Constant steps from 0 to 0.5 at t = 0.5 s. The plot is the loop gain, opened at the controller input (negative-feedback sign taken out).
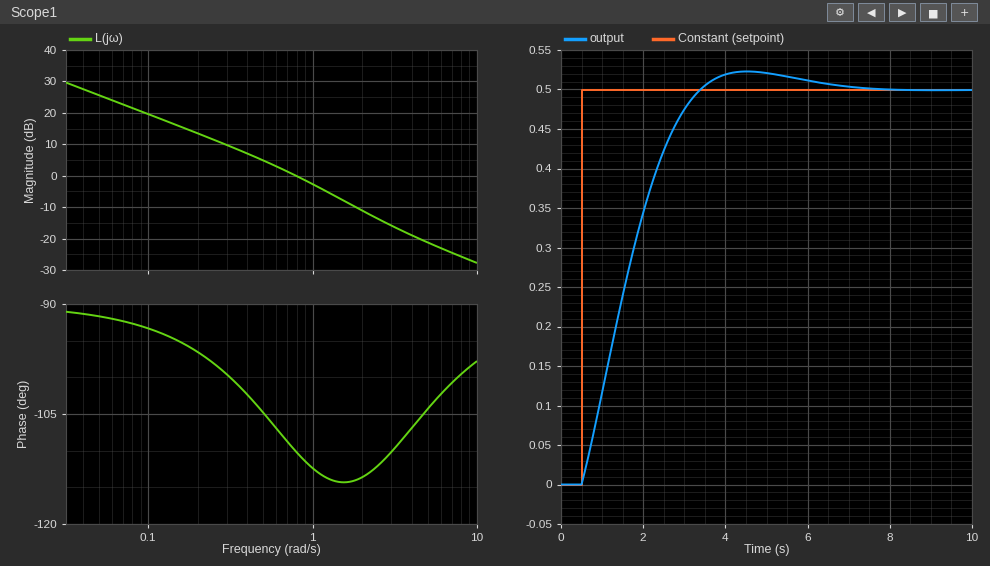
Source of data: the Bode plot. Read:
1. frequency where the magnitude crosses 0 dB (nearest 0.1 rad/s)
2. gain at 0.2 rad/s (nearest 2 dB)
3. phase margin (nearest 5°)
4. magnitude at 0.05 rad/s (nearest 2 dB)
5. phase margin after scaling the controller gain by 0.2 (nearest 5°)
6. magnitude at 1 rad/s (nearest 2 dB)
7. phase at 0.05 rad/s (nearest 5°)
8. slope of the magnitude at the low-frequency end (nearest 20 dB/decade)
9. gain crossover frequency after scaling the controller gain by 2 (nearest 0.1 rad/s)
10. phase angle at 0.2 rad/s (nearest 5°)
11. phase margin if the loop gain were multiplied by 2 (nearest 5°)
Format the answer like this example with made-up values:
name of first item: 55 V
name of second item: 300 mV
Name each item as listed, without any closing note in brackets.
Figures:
frequency where the magnitude crosses 0 dB: 0.8 rad/s
gain at 0.2 rad/s: 14 dB
phase margin: 70°
magnitude at 0.05 rad/s: 26 dB
phase margin after scaling the controller gain by 0.2: 85°
magnitude at 1 rad/s: -2 dB
phase at 0.05 rad/s: -90°
slope of the magnitude at the low-frequency end: -20 dB/decade
gain crossover frequency after scaling the controller gain by 2: 1.3 rad/s
phase angle at 0.2 rad/s: -95°
phase margin if the loop gain were multiplied by 2: 65°
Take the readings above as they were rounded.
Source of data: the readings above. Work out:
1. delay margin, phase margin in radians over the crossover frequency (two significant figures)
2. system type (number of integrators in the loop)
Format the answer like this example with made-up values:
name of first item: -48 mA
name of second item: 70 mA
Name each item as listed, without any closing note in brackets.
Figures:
delay margin, phase margin in radians over the crossover frequency: 1.5 s
system type: 1
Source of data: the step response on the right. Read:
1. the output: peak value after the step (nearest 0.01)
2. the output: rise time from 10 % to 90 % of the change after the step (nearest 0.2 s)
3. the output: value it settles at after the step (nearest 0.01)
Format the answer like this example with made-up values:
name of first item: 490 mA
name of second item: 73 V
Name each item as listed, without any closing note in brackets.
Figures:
the output: peak value after the step: 0.52
the output: rise time from 10 % to 90 % of the change after the step: 2.0 s
the output: value it settles at after the step: 0.50
